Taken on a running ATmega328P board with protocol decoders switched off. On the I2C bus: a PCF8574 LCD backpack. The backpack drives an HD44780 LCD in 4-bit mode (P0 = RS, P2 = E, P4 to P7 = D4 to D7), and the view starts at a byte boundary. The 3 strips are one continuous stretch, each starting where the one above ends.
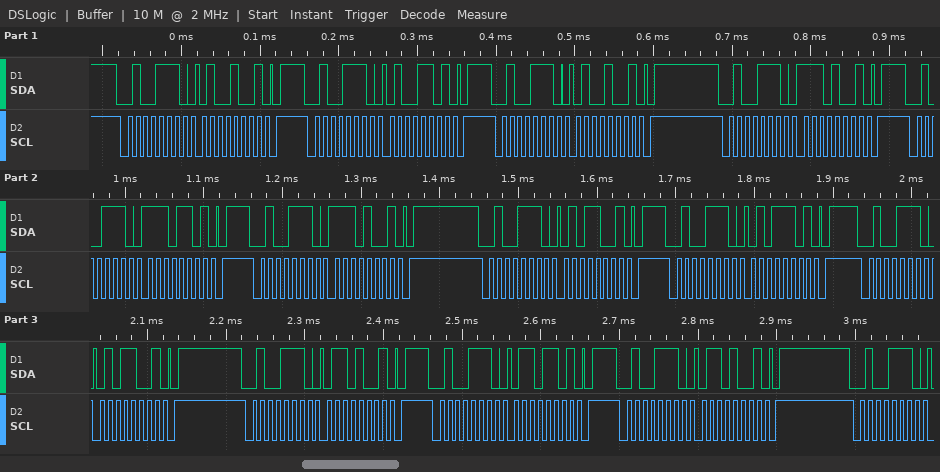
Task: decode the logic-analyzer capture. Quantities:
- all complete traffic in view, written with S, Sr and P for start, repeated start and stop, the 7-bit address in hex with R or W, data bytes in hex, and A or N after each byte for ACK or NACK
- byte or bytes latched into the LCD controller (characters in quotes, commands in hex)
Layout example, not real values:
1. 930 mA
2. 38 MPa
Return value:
1. S 27W A 49 A P S 27W A 4D A P S 27W A 49 A P S 27W A E9 A P S 27W A ED A P S 27W A E9 A P S 27W A 59 A P S 27W A 5D A P S 27W A 59 A P S 27W A 69 A P S 27W A 6D A P S 27W A 69 A P S 27W A
2. 'N' 'V'
